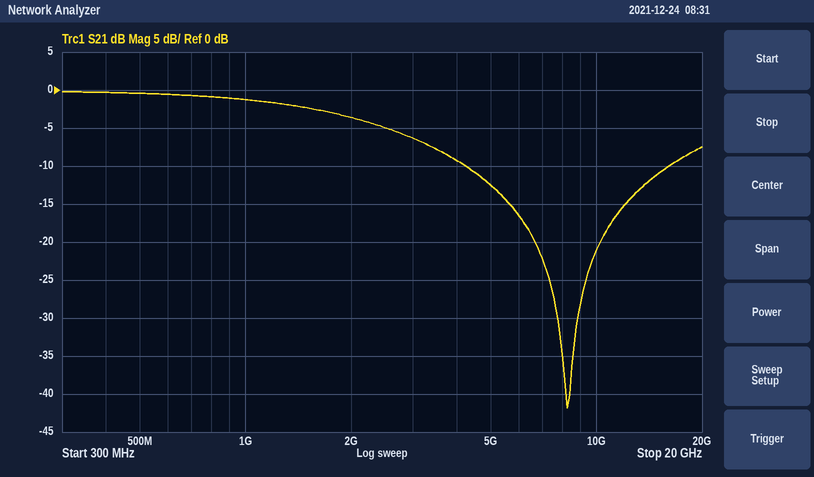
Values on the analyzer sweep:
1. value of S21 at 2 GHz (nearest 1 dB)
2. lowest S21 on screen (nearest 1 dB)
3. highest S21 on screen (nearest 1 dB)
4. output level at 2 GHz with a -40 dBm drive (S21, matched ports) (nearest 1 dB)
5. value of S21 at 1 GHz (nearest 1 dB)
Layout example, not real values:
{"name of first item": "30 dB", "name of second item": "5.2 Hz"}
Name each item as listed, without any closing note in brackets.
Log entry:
{"value of S21 at 2 GHz": "-4 dB", "lowest S21 on screen": "-42 dB", "highest S21 on screen": "0 dB", "output level at 2 GHz with a -40 dBm drive (S21, matched ports)": "-44 dBm", "value of S21 at 1 GHz": "-1 dB"}
